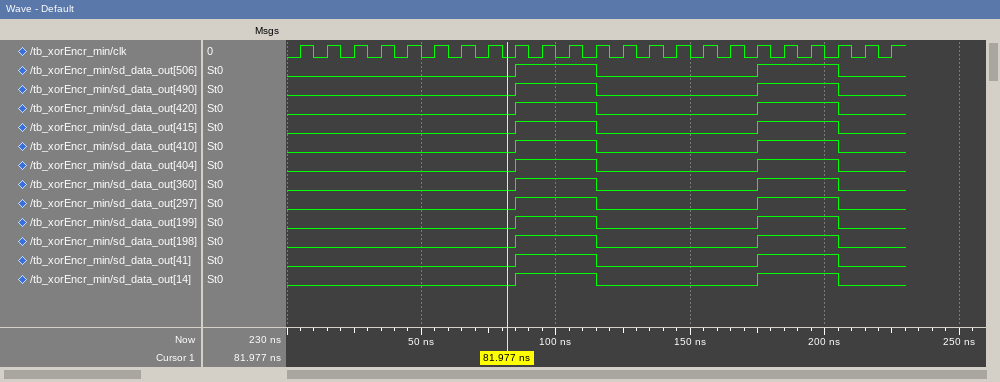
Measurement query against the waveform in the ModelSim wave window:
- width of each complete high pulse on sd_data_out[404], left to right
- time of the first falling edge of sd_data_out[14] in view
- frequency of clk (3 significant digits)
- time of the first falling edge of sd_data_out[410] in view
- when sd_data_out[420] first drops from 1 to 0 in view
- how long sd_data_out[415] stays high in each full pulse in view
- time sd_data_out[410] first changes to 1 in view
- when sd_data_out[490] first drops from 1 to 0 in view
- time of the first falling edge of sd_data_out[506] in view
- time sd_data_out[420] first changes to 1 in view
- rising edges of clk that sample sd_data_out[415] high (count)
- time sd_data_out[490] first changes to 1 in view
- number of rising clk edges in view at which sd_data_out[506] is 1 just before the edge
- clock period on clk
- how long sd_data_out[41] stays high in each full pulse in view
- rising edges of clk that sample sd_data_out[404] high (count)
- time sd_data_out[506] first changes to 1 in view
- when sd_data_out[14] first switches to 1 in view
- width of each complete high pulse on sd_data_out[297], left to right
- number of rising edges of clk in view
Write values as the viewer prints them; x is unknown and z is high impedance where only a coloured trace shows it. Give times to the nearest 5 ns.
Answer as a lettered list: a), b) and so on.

a) 30 ns, 30 ns
b) 115 ns
c) 100 MHz
d) 115 ns
e) 115 ns
f) 30 ns, 30 ns
g) 85 ns
h) 115 ns
i) 115 ns
j) 85 ns
k) 6
l) 85 ns
m) 6
n) 10 ns
o) 30 ns, 30 ns
p) 6
q) 85 ns
r) 85 ns
s) 30 ns, 30 ns
t) 23
